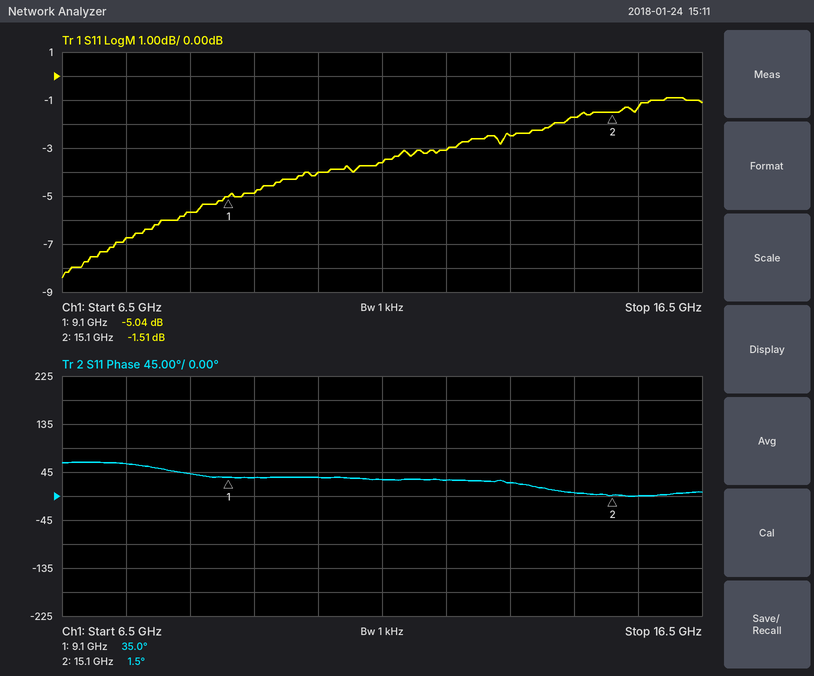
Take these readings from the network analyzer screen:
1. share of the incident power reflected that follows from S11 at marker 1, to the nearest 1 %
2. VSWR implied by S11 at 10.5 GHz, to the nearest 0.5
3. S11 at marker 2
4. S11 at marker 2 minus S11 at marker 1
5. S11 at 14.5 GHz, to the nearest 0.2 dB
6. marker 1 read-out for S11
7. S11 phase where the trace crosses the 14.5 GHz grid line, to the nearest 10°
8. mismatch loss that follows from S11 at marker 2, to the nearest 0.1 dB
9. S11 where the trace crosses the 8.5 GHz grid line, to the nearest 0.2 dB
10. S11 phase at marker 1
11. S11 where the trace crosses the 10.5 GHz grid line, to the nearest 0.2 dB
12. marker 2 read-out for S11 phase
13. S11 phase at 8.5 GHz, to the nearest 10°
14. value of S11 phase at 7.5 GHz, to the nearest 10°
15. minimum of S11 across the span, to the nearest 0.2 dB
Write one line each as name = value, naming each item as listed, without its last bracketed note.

share of the incident power reflected that follows from S11 at marker 1, to the nearest 1 % = 31 %
VSWR implied by S11 at 10.5 GHz, to the nearest 0.5 = 4.5
S11 at marker 2 = -1.51 dB
S11 at marker 2 minus S11 at marker 1 = 3.53 dB
S11 at 14.5 GHz, to the nearest 0.2 dB = -1.8 dB
marker 1 read-out for S11 = -5.04 dB
S11 phase where the trace crosses the 14.5 GHz grid line, to the nearest 10° = 10°
mismatch loss that follows from S11 at marker 2, to the nearest 0.1 dB = 5.3 dB
S11 where the trace crosses the 8.5 GHz grid line, to the nearest 0.2 dB = -5.6 dB
S11 phase at marker 1 = 35.0°
S11 where the trace crosses the 10.5 GHz grid line, to the nearest 0.2 dB = -4.0 dB
marker 2 read-out for S11 phase = 1.5°
S11 phase at 8.5 GHz, to the nearest 10° = 40°
value of S11 phase at 7.5 GHz, to the nearest 10° = 60°
minimum of S11 across the span, to the nearest 0.2 dB = -8.4 dB
